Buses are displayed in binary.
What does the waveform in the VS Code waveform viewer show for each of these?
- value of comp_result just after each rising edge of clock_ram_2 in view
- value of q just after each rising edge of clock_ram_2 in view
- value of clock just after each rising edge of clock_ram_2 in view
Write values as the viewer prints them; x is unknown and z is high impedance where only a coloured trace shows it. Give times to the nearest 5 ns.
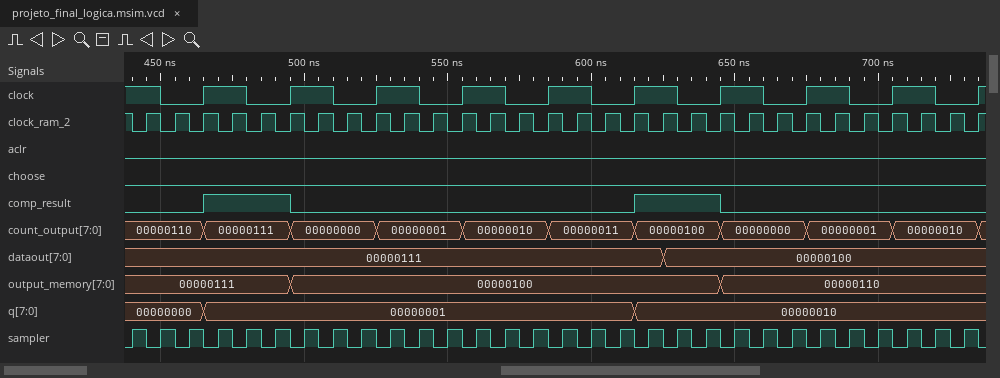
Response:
0 0 1 1 1 0 0 0 0 0 0 0 0 0 0 0 0 1 1 1 0 0 0 0 0 0 0 0 0 0
00000000, 00000000, 00000001, 00000001, 00000001, 00000001, 00000001, 00000001, 00000001, 00000001, 00000001, 00000001, 00000001, 00000001, 00000001, 00000001, 00000001, 00000010, 00000010, 00000010, 00000010, 00000010, 00000010, 00000010, 00000010, 00000010, 00000010, 00000010, 00000010, 00000010
1 0 1 1 0 1 1 0 1 1 0 1 1 0 1 1 0 1 1 0 1 1 0 1 1 0 1 1 0 1
